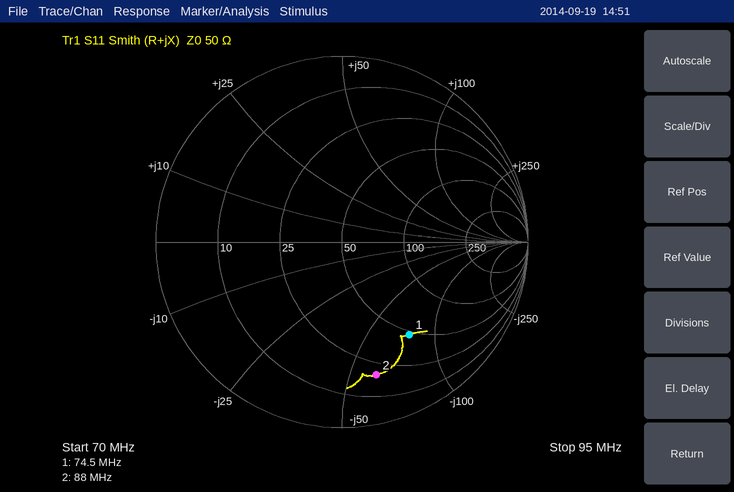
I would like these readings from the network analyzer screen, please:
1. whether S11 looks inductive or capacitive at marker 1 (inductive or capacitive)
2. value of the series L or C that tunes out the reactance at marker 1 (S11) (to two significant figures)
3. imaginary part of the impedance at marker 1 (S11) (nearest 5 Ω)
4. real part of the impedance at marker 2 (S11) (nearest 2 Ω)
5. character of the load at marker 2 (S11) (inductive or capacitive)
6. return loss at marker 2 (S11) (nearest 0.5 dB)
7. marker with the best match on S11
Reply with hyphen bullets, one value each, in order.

- capacitive
- 160 nH
- -75 Ω
- 20 Ω
- capacitive
- 2.5 dB
- marker 1
